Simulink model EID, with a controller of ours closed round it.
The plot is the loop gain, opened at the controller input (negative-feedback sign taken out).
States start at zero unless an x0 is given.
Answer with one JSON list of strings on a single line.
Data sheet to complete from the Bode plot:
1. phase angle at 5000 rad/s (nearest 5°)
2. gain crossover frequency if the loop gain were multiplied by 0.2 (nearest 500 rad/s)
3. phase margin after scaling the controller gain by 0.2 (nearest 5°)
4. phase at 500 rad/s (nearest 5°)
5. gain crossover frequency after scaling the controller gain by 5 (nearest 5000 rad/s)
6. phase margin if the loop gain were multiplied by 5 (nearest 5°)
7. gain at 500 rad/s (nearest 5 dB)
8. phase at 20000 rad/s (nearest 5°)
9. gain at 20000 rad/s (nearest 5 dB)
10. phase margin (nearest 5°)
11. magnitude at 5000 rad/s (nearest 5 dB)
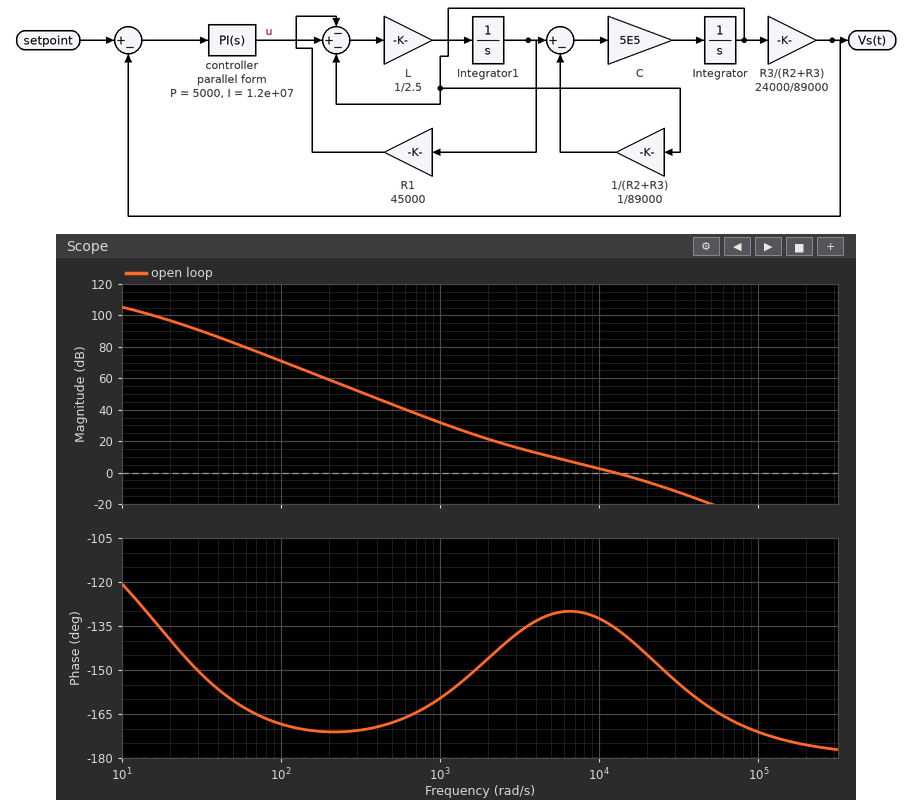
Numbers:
["-130°", "3500 rad/s", "45°", "-170°", "35000 rad/s", "25°", "45 dB", "-145°", "-5 dB", "45°", "10 dB"]
